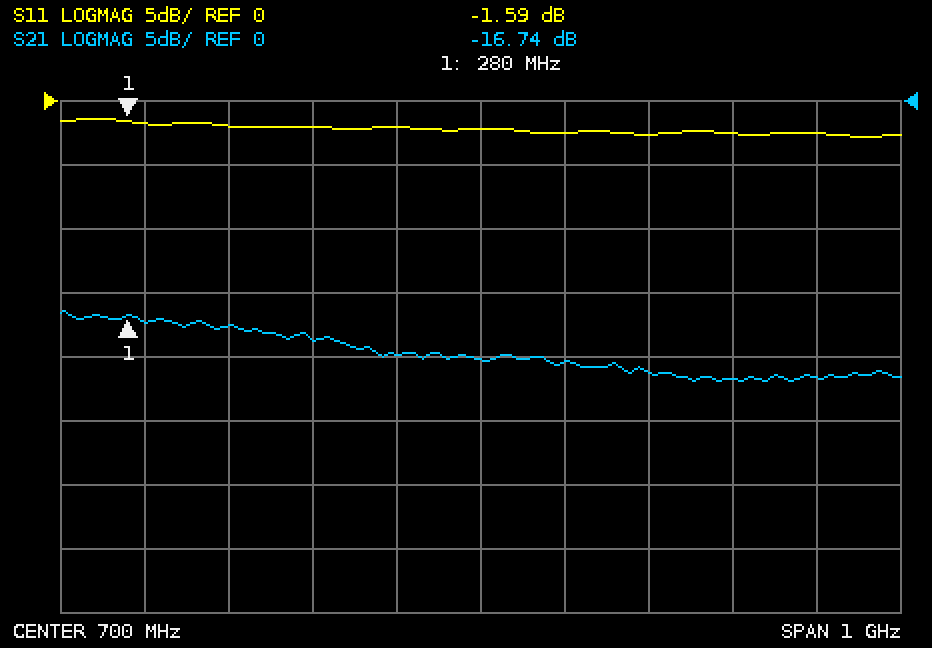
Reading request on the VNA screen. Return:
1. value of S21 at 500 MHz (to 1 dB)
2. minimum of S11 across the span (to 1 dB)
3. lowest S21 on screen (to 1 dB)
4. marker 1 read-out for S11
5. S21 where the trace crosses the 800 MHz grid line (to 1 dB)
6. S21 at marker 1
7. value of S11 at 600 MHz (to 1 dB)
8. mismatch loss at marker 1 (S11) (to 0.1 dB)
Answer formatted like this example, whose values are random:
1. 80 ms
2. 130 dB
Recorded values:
1. -19 dB
2. -3 dB
3. -22 dB
4. -1.59 dB
5. -20 dB
6. -16.74 dB
7. -2 dB
8. 5.1 dB
